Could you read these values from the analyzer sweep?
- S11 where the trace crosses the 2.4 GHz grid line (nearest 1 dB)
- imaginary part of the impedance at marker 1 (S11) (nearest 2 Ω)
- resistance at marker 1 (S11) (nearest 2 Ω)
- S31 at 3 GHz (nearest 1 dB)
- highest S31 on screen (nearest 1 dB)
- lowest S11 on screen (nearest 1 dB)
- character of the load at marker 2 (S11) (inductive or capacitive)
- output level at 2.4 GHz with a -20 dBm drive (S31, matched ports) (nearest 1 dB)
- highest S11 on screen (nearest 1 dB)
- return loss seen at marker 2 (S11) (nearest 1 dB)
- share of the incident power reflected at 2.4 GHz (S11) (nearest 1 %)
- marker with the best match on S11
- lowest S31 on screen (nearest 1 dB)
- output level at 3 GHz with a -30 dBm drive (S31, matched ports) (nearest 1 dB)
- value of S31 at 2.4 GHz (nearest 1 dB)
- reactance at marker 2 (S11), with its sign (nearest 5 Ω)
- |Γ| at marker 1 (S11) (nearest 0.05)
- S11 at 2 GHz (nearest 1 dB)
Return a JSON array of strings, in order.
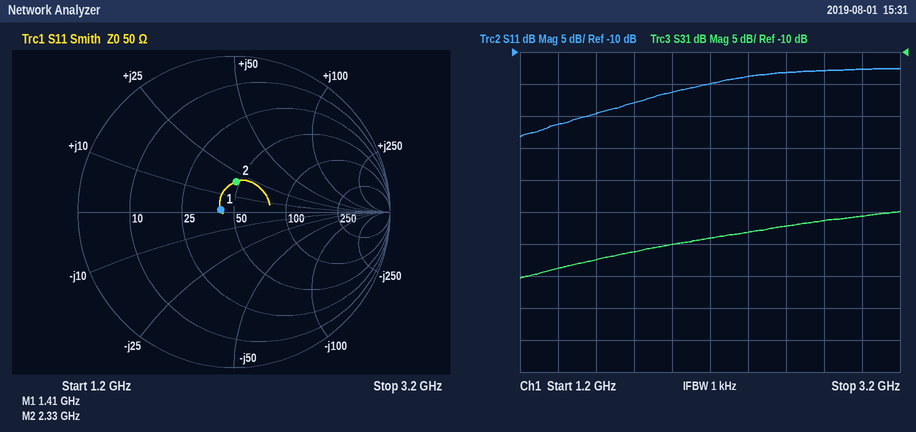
["-14 dB", "+2 Ω", "42 Ω", "-36 dB", "-35 dB", "-23 dB", "inductive", "-58 dBm", "-13 dB", "14 dB", "4 %", "marker 1", "-45 dB", "-66 dBm", "-38 dB", "+20 Ω", "0.10", "-16 dB"]
